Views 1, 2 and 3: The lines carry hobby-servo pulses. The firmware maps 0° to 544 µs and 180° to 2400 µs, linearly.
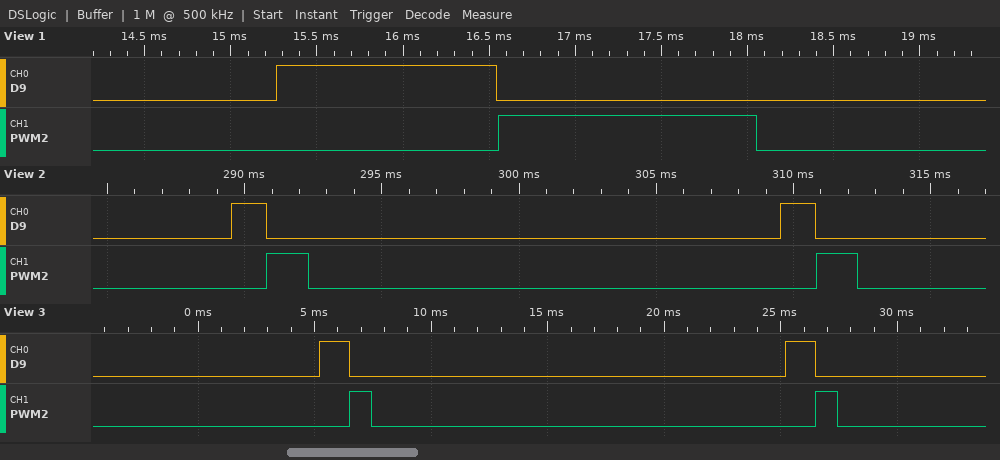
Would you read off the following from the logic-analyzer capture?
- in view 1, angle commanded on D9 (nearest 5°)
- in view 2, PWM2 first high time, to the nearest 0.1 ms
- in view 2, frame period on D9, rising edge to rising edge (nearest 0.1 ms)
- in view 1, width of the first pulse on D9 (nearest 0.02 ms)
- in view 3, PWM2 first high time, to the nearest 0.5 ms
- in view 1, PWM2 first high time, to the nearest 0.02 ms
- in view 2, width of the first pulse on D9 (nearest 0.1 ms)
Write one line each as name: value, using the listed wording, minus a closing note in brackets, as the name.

in view 1, angle commanded on D9: 70°
in view 2, PWM2 first high time, to the nearest 0.1 ms: 1.5 ms
in view 2, frame period on D9, rising edge to rising edge: 20.0 ms
in view 1, width of the first pulse on D9: 1.28 ms
in view 3, PWM2 first high time, to the nearest 0.5 ms: 1.0 ms
in view 1, PWM2 first high time, to the nearest 0.02 ms: 1.50 ms
in view 2, width of the first pulse on D9: 1.3 ms
